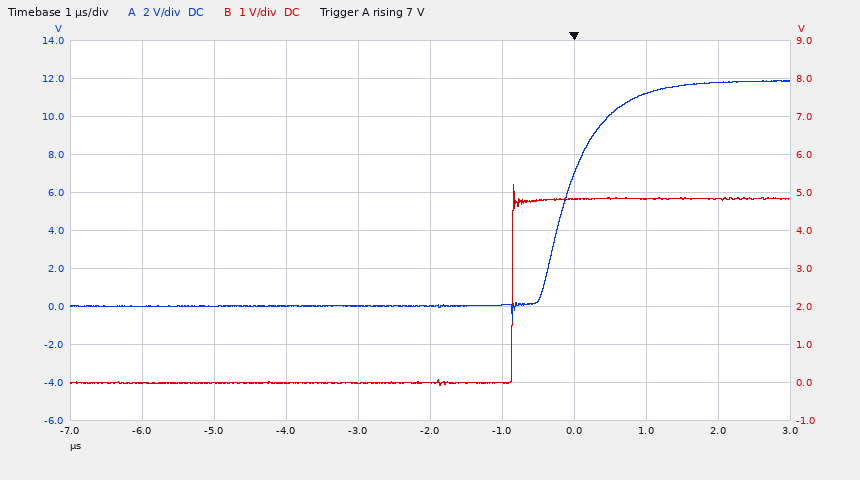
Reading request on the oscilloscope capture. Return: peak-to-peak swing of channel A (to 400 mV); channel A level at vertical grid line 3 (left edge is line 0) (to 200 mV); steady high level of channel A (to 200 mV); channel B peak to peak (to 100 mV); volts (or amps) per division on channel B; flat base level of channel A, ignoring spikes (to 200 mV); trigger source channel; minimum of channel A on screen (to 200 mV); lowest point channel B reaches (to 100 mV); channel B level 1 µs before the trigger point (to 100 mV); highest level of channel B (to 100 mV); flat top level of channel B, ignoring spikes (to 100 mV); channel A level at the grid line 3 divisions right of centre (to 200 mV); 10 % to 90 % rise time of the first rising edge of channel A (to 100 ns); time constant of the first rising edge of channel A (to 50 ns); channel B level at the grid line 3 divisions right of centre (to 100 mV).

12.8 V
0.0 V
11.8 V
5.3 V
1 V
0.0 V
channel A
-800 mV
-100 mV
0.0 V
5.2 V
4.8 V
11.2 V
1.1 µs
500 ns
4.8 V
